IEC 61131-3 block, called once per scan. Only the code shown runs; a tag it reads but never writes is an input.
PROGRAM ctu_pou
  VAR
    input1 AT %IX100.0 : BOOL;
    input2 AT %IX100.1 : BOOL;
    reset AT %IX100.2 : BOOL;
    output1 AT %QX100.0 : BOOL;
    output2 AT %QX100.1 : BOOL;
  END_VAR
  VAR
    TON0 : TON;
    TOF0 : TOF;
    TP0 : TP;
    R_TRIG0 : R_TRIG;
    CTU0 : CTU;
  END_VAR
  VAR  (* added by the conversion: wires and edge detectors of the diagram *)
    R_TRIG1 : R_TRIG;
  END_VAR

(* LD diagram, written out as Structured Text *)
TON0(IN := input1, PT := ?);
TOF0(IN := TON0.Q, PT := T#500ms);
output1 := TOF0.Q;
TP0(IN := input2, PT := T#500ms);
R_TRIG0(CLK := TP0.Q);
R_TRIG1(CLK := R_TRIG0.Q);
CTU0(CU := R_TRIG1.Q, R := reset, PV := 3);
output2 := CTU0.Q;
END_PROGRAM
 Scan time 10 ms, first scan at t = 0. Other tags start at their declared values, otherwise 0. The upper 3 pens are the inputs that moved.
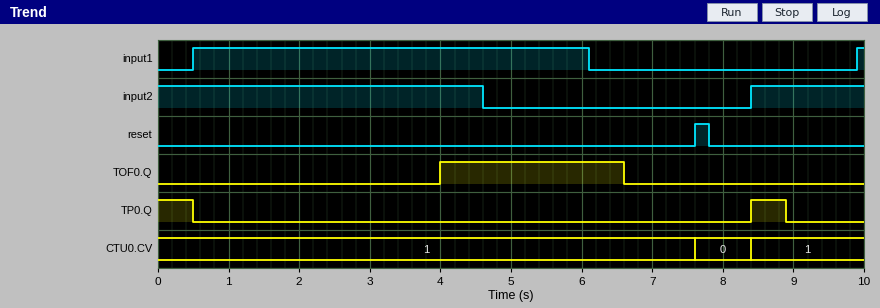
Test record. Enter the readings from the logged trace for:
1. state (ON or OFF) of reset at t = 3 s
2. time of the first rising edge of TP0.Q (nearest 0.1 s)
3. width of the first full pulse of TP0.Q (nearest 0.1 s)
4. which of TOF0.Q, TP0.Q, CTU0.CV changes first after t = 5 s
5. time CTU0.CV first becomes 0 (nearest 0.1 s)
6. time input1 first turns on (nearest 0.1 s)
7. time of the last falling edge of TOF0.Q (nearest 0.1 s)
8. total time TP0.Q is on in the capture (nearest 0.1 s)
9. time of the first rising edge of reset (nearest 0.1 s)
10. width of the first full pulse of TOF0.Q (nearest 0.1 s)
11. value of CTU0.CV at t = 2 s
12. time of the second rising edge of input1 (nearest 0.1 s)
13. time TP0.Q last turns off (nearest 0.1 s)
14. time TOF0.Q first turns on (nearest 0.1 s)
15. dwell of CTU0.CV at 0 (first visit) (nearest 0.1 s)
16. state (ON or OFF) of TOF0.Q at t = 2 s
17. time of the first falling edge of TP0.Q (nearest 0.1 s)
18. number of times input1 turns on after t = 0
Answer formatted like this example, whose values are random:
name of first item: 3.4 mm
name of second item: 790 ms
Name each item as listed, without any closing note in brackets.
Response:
state (ON or OFF) of reset at t = 3 s: OFF
time of the first rising edge of TP0.Q: 8.4 s
width of the first full pulse of TP0.Q: 0.5 s
which of TOF0.Q, TP0.Q, CTU0.CV changes first after t = 5 s: TOF0.Q
time CTU0.CV first becomes 0: 7.6 s
time input1 first turns on: 0.5 s
time of the last falling edge of TOF0.Q: 6.6 s
total time TP0.Q is on in the capture: 1.0 s
time of the first rising edge of reset: 7.6 s
width of the first full pulse of TOF0.Q: 2.6 s
value of CTU0.CV at t = 2 s: 1
time of the second rising edge of input1: 9.9 s
time TP0.Q last turns off: 8.9 s
time TOF0.Q first turns on: 4.0 s
dwell of CTU0.CV at 0 (first visit): 0.8 s
state (ON or OFF) of TOF0.Q at t = 2 s: OFF
time of the first falling edge of TP0.Q: 0.5 s
number of times input1 turns on after t = 0: 2
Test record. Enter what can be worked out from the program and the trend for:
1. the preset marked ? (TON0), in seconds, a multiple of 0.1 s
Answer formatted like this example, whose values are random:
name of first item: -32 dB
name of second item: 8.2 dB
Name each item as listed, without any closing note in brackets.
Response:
the preset marked ? (TON0), in seconds, a multiple of 0.1 s: 3.5 s
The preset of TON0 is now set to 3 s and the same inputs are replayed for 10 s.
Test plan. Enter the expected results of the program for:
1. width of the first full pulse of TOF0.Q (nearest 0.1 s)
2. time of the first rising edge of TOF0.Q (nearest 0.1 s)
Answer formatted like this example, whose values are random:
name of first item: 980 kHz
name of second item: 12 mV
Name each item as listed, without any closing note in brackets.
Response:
width of the first full pulse of TOF0.Q: 3.1 s
time of the first rising edge of TOF0.Q: 3.5 s
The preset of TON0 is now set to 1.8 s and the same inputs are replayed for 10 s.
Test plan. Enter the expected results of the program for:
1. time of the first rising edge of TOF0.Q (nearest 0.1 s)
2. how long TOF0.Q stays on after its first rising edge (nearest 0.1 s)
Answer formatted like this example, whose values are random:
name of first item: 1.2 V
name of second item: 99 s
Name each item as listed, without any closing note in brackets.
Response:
time of the first rising edge of TOF0.Q: 2.3 s
how long TOF0.Q stays on after its first rising edge: 4.3 s
